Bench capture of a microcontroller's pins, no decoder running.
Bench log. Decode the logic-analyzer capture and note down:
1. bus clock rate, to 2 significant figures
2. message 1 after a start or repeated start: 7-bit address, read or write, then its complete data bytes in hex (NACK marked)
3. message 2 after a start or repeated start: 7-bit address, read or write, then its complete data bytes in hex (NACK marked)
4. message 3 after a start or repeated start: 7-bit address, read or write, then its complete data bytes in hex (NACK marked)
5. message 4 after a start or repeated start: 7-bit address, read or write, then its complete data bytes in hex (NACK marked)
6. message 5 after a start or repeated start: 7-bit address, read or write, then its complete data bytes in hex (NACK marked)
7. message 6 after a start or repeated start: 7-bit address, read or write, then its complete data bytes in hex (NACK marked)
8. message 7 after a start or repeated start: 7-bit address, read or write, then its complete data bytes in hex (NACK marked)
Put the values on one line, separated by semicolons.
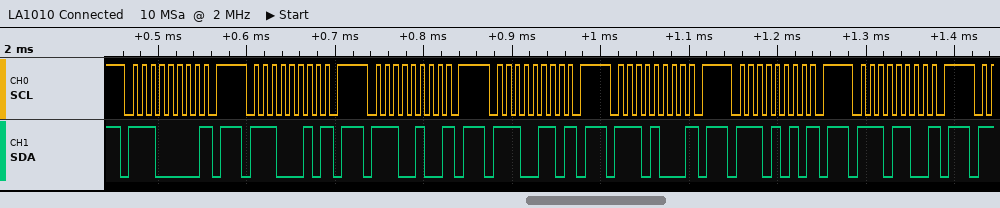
100 kHz; 0x70 write NACK; 0x71 write NACK; 0x72 write NACK; 0x73 write NACK; 0x74 write NACK; 0x75 write NACK; 0x76 write NACK
